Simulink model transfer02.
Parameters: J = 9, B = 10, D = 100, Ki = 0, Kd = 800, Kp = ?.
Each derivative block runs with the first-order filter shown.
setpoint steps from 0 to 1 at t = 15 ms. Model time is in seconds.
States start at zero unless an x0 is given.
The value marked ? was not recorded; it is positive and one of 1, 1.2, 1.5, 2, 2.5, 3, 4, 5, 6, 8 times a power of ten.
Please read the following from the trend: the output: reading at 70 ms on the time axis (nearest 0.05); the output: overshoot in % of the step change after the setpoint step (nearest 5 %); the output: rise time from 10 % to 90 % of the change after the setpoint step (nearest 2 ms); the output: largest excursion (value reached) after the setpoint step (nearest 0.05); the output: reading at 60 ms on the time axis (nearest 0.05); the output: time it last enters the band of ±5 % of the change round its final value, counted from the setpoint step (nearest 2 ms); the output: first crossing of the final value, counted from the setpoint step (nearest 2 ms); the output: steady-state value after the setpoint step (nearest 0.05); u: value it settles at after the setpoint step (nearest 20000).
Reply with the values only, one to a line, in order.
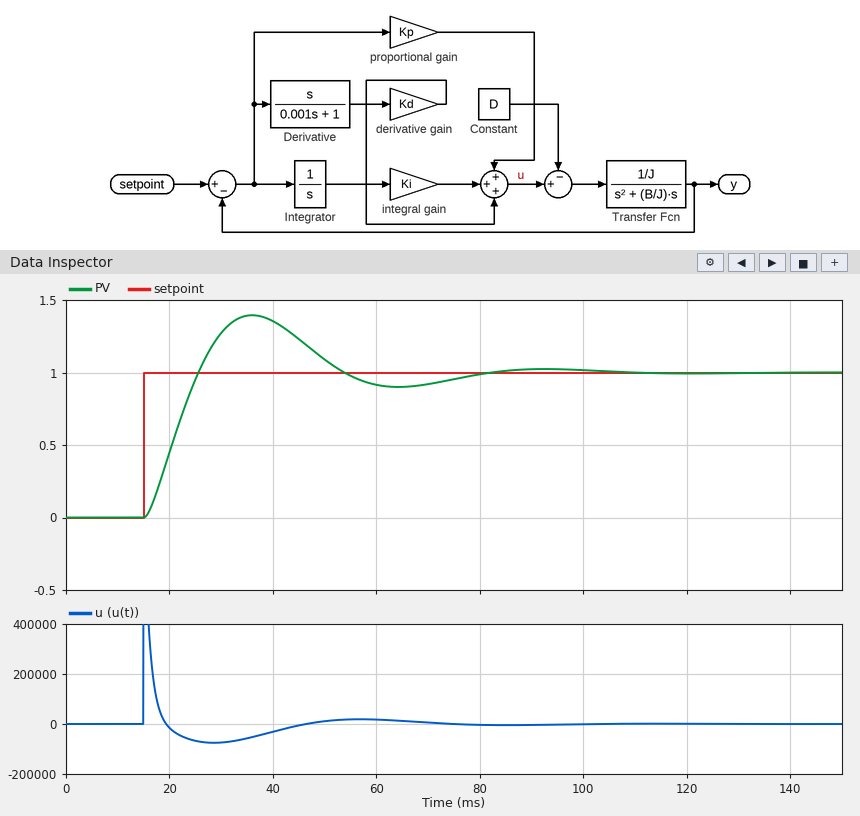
0.90
40 %
8 ms
1.40
0.90
60 ms
10 ms
1.00
0
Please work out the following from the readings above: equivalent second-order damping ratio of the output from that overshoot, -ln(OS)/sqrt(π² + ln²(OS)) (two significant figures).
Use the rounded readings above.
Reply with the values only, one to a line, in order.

0.28
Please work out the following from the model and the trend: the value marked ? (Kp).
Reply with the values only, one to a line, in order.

120000
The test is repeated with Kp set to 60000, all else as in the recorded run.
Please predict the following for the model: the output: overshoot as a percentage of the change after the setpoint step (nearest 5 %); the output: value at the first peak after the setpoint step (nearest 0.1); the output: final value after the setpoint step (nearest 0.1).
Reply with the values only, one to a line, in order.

30 %
1.3
1.0
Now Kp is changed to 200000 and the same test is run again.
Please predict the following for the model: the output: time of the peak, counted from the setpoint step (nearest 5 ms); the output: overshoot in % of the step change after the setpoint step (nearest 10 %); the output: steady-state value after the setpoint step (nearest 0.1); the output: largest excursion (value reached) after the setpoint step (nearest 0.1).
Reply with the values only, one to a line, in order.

15 ms
50 %
1.0
1.5
